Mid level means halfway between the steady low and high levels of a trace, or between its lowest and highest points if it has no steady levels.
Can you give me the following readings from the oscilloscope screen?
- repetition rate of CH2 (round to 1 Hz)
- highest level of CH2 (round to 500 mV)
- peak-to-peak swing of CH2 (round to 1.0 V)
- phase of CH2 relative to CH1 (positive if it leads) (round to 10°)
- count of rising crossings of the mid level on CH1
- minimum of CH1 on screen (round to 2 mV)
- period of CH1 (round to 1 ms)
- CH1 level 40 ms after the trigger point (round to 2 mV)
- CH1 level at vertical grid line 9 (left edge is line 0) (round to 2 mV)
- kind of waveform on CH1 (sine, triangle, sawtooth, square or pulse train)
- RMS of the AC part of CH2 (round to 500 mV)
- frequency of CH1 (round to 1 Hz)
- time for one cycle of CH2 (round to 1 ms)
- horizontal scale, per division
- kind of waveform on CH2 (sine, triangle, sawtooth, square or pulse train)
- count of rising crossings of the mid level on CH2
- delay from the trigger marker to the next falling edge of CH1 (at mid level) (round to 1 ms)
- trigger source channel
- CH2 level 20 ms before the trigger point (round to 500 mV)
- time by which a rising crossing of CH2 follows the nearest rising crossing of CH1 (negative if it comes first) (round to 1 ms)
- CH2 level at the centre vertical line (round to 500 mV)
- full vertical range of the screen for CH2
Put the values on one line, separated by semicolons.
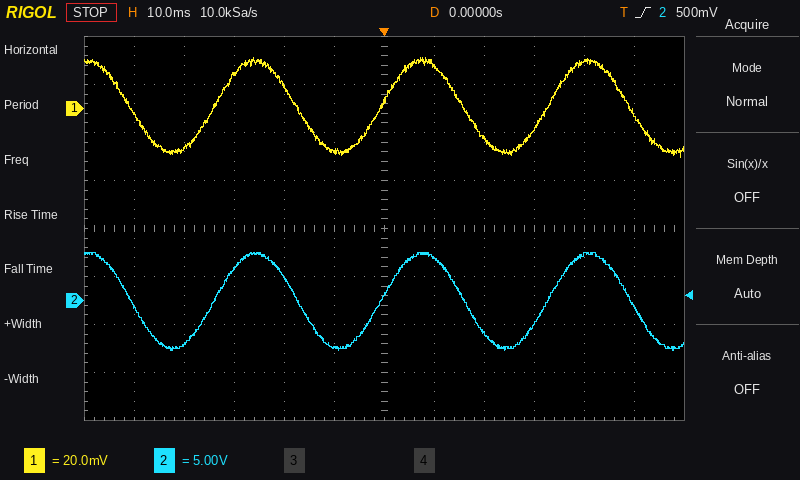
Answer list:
30 Hz; 5.0 V; 10.0 V; 0°; 3; -20 mV; 33 ms; 20 mV; -8 mV; sine; 3.5 V; 30 Hz; 33 ms; 10 ms; sine; 3; 16 ms; CH2; 2.5 V; 0 ms; 500 mV; 40 V
